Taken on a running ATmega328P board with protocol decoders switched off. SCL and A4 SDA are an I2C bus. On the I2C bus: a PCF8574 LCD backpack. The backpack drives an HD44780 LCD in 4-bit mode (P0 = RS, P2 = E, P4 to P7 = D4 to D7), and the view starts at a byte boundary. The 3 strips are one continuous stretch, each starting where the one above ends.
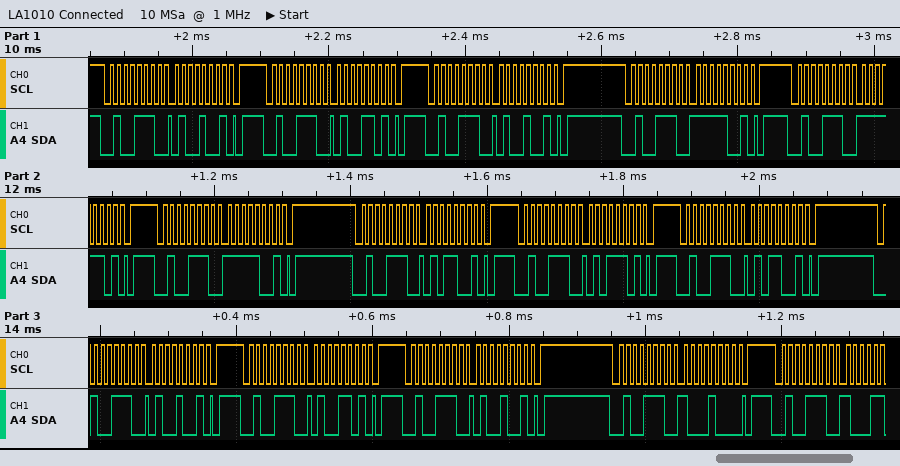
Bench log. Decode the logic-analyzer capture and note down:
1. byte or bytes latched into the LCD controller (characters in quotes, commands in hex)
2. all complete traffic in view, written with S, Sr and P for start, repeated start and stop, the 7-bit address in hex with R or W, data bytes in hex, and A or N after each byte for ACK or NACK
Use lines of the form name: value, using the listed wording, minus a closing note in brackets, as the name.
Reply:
byte or bytes latched into the LCD controller: 'O' 'T'
all complete traffic in view, written with S, Sr and P for start, repeated start and stop, the 7-bit address in hex with R or W, data bytes in hex, and A or N after each byte for ACK or NACK: S 27W A 49 A P S 27W A 4D A P S 27W A 49 A P S 27W A F9 A P S 27W A FD A P S 27W A F9 A P S 27W A 59 A P S 27W A 5D A P S 27W A 59 A P S 27W A 49 A P S 27W A 4D A P S 27W A 49 A P S 27W A 88 A P S 27W A
